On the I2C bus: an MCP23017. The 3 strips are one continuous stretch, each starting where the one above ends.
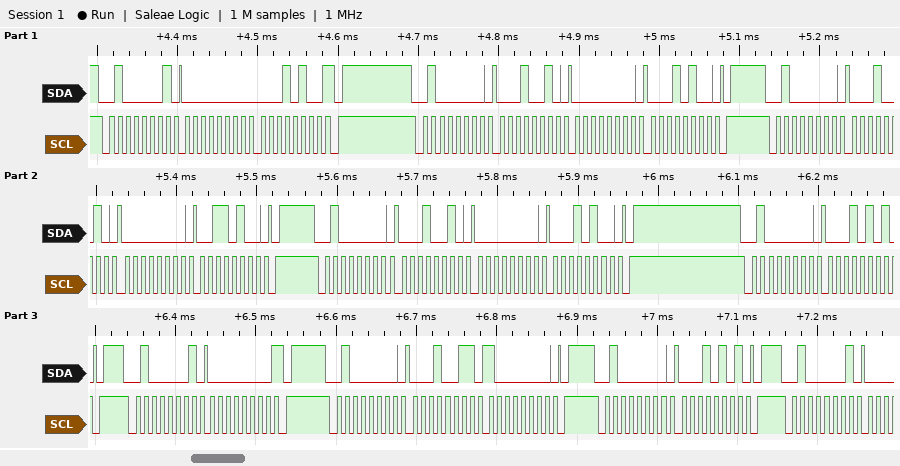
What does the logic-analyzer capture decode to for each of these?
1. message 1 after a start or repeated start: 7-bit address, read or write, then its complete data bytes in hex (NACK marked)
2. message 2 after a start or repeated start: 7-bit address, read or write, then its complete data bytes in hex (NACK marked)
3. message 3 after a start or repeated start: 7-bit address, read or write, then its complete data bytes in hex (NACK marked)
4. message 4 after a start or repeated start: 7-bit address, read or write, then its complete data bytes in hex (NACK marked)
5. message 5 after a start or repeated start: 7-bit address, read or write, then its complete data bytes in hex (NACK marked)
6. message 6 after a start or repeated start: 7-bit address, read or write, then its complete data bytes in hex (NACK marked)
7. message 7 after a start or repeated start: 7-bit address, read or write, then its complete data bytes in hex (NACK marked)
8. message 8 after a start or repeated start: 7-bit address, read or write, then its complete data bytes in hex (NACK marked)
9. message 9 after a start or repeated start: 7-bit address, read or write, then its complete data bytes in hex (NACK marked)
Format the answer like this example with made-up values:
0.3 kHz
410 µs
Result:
0x20 read: 00 14 NACK
0x20 write: 12 00 14
0x20 write: 12 00 34
0x20 write: 12 00 14
0x20 write: 15
0x20 read: 00 NACK
0x20 write: 13 80
0x20 write: 15
0x20 read
